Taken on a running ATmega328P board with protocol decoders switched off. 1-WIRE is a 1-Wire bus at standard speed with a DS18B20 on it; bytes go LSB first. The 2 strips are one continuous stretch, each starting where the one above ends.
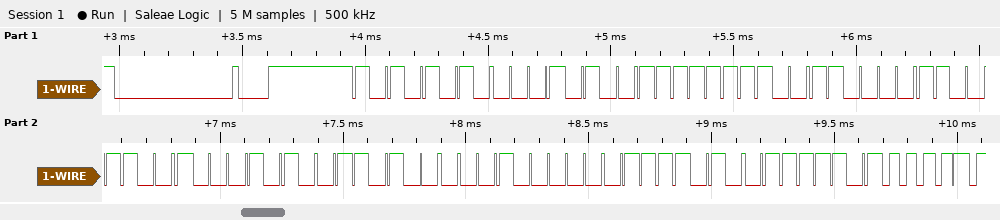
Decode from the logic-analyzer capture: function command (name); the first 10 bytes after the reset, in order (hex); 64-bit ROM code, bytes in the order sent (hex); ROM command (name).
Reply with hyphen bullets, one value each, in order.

- Read Scratchpad
- 55 28 FF 0C 33 51 16 04 5E BE
- 28 FF 0C 33 51 16 04 5E
- Match ROM
